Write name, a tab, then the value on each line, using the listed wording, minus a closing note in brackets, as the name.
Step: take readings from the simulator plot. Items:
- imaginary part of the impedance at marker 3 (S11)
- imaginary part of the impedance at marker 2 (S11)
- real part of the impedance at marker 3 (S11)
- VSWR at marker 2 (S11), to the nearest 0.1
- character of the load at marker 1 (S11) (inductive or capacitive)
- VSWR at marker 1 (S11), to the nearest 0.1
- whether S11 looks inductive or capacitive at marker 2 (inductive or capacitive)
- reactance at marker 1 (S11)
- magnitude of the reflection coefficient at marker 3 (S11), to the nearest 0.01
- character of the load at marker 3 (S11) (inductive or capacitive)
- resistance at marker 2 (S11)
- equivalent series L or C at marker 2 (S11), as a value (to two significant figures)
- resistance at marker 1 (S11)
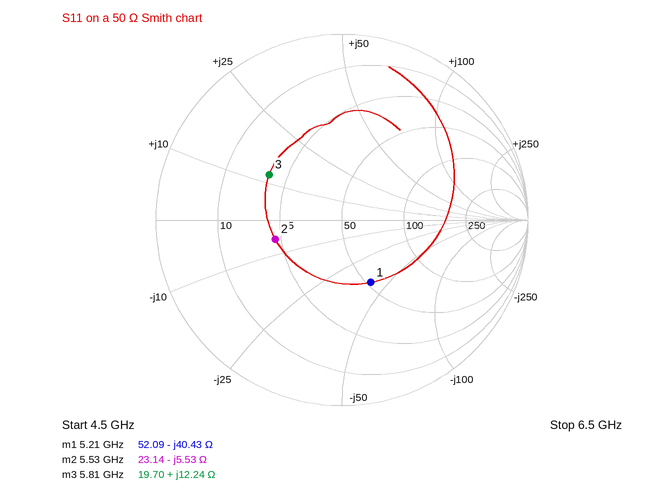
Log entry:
imaginary part of the impedance at marker 3	+12.24 Ω
imaginary part of the impedance at marker 2	-5.53 Ω
real part of the impedance at marker 3	19.70 Ω
VSWR at marker 2 (S11), to the nearest 0.1	2.2
character of the load at marker 1 (S11)	capacitive
VSWR at marker 1 (S11), to the nearest 0.1	2.2
whether S11 looks inductive or capacitive at marker 2	capacitive
reactance at marker 1	-40.43 Ω
magnitude of the reflection coefficient at marker 3 (S11), to the nearest 0.01	0.46
character of the load at marker 3 (S11)	inductive
resistance at marker 2	23.14 Ω
equivalent series L or C at marker 2 (S11), as a value	5.2 pF
resistance at marker 1	52.09 Ω
